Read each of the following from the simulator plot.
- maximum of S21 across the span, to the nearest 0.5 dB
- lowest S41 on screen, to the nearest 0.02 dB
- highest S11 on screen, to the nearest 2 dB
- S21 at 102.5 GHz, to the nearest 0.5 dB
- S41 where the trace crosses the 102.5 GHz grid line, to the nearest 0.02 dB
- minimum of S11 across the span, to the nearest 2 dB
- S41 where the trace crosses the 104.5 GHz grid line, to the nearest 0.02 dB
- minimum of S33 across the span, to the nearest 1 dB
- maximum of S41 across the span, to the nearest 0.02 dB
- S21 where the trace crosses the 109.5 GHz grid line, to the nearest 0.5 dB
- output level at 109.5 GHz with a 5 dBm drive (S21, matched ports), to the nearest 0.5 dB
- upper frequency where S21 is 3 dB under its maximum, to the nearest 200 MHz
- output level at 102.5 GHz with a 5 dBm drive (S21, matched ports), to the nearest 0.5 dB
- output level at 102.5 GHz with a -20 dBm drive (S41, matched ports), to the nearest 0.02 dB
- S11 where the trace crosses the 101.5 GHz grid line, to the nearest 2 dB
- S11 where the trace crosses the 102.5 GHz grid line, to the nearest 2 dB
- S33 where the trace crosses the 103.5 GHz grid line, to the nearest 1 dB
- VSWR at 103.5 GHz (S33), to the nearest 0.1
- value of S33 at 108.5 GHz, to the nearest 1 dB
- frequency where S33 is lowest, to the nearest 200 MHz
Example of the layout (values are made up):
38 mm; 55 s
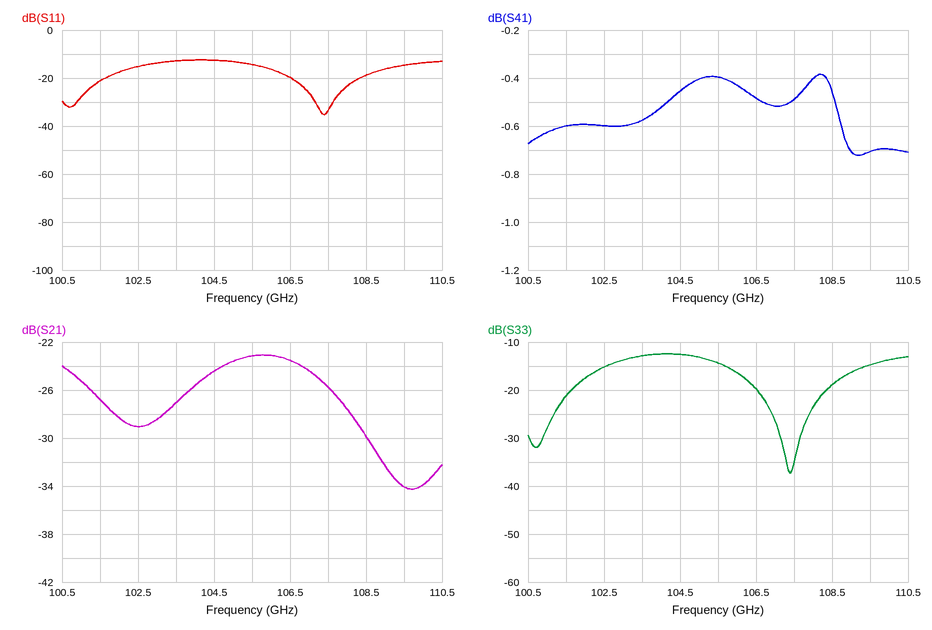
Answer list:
-23.0 dB; -0.72 dB; -12 dB; -29.0 dB; -0.60 dB; -36 dB; -0.46 dB; -37 dB; -0.38 dB; -34.0 dB; -29.0 dBm; 107.6 GHz; -24.0 dBm; -20.60 dBm; -22 dB; -16 dB; -13 dB; 1.6; -19 dB; 107.4 GHz
